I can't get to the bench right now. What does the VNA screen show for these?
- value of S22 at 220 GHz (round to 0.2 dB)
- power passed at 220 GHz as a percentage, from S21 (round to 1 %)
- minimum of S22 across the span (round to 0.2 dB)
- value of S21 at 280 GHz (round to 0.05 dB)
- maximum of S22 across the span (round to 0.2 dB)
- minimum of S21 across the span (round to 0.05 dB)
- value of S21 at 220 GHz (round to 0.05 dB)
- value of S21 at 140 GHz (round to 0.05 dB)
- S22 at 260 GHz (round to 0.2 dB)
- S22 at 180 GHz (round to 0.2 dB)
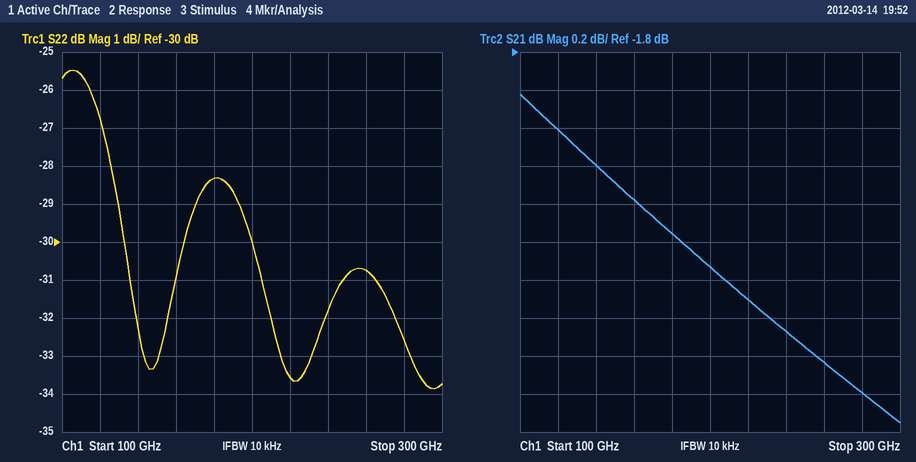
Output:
-33.6 dB
49 %
-33.8 dB
-3.60 dB
-25.4 dB
-3.75 dB
-3.10 dB
-2.40 dB
-30.8 dB
-28.4 dB
